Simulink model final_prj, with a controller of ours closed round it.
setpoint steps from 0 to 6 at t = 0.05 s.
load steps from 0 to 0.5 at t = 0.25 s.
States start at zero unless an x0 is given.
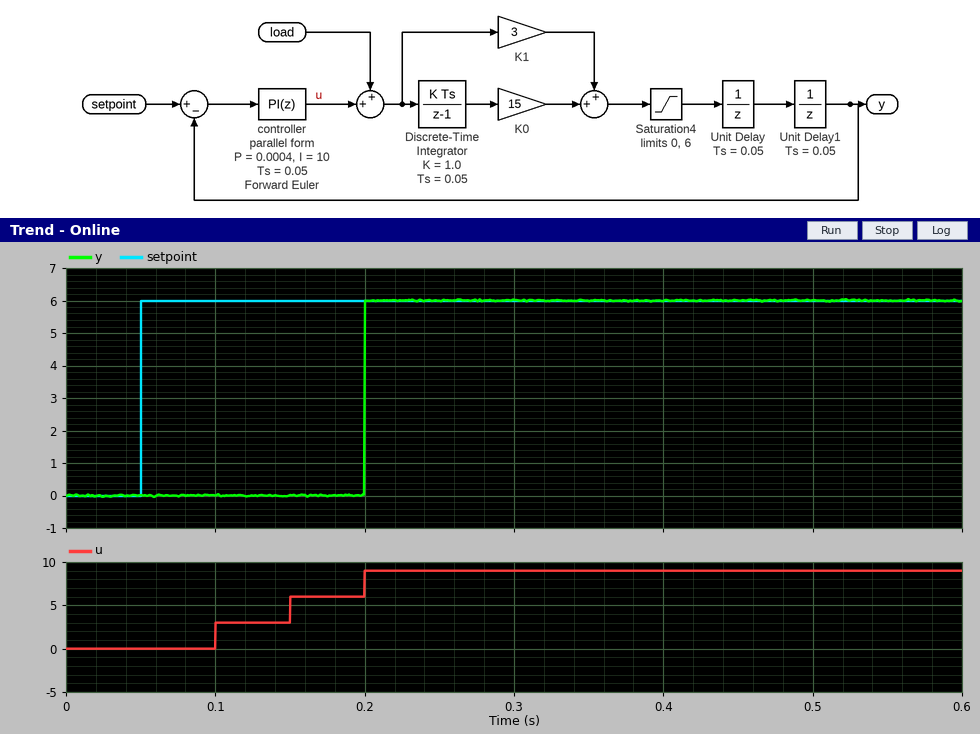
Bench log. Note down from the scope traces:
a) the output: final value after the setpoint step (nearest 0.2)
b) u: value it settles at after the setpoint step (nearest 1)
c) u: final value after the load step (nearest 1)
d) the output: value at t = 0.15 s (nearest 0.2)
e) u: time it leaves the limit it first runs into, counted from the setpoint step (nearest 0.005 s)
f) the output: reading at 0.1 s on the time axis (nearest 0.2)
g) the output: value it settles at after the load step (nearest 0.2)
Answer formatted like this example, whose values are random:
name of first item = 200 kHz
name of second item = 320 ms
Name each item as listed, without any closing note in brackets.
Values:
the output: final value after the setpoint step = 6.0
u: value it settles at after the setpoint step = 9
u: final value after the load step = 9
the output: value at t = 0.15 s = 0.0
u: time it leaves the limit it first runs into, counted from the setpoint step = 0.050 s
the output: reading at 0.1 s on the time axis = 0.0
the output: value it settles at after the load step = 6.0
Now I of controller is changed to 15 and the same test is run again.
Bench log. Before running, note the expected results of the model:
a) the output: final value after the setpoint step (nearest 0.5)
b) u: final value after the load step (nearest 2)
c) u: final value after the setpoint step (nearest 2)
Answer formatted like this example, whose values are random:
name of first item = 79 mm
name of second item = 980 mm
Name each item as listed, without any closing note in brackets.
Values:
the output: final value after the setpoint step = 6.0
u: final value after the load step = 14
u: final value after the setpoint step = 14
